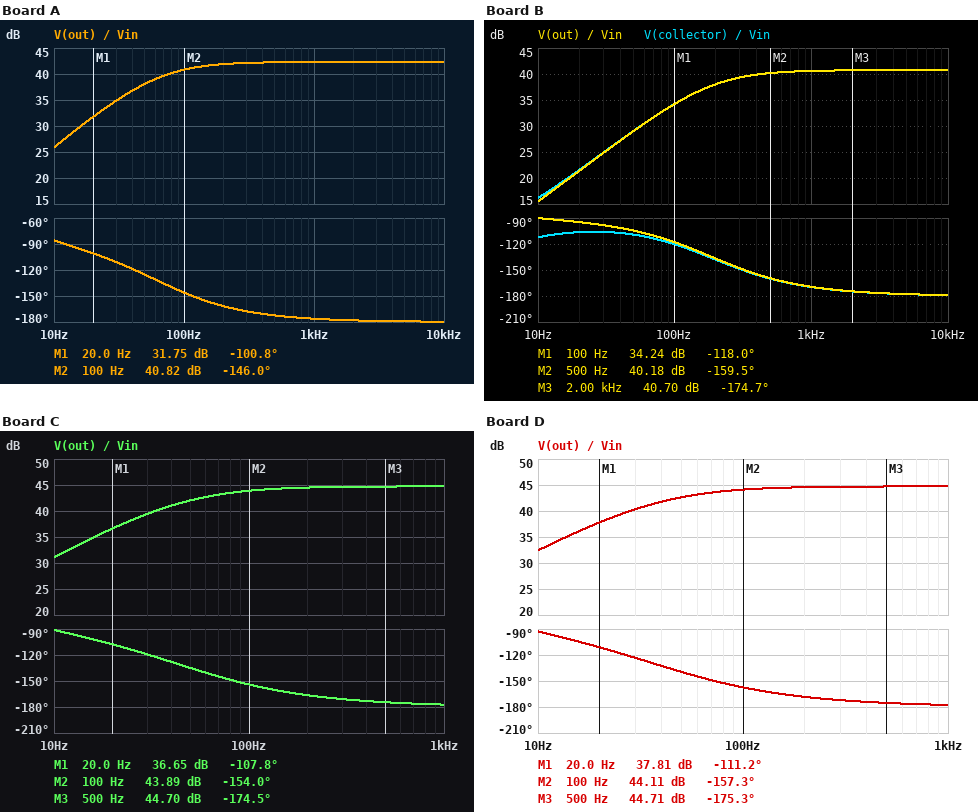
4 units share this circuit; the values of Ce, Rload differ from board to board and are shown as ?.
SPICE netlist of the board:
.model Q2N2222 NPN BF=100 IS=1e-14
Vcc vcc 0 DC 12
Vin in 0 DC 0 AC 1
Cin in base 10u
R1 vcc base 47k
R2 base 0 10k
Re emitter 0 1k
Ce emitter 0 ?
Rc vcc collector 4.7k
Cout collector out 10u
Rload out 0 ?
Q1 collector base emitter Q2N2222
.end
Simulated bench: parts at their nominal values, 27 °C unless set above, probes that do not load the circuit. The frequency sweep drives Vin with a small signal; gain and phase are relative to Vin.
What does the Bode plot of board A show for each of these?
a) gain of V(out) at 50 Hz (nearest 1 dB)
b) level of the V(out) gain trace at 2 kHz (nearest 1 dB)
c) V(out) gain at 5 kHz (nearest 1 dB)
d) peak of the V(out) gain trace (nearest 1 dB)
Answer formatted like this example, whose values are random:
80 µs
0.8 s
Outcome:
38 dB
42 dB
42 dB
42 dB
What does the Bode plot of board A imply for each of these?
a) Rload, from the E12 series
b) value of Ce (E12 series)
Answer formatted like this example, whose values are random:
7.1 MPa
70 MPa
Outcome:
5.6 kΩ
150 µF
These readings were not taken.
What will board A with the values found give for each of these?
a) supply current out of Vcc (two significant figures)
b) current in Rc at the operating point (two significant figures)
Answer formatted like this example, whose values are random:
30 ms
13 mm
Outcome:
1.5 mA
1.3 mA
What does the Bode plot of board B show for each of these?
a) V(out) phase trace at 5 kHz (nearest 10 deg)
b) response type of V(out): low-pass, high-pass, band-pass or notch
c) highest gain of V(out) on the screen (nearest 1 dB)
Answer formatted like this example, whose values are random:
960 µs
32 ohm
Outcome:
-180 deg
high-pass
41 dB
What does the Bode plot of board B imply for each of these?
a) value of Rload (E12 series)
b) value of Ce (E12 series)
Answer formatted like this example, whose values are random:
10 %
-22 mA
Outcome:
3.9 kΩ
47 µF
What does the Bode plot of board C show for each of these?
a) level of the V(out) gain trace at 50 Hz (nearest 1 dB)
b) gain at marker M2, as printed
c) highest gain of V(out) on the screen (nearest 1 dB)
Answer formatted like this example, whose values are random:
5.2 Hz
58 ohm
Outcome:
42 dB
43.89 dB
45 dB
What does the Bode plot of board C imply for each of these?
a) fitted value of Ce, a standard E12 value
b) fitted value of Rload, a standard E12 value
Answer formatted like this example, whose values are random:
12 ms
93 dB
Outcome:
220 µF
12 kΩ
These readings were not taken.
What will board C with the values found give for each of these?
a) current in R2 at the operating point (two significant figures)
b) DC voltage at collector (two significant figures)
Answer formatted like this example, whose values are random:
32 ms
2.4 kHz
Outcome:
200 µA
5.8 V
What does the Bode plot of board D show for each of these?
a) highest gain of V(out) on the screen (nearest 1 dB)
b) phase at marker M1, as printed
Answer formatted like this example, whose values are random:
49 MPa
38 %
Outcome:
45 dB
-111.2 deg
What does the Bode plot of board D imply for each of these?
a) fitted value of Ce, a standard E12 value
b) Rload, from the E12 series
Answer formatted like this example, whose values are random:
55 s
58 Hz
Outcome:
270 µF
12 kΩ
